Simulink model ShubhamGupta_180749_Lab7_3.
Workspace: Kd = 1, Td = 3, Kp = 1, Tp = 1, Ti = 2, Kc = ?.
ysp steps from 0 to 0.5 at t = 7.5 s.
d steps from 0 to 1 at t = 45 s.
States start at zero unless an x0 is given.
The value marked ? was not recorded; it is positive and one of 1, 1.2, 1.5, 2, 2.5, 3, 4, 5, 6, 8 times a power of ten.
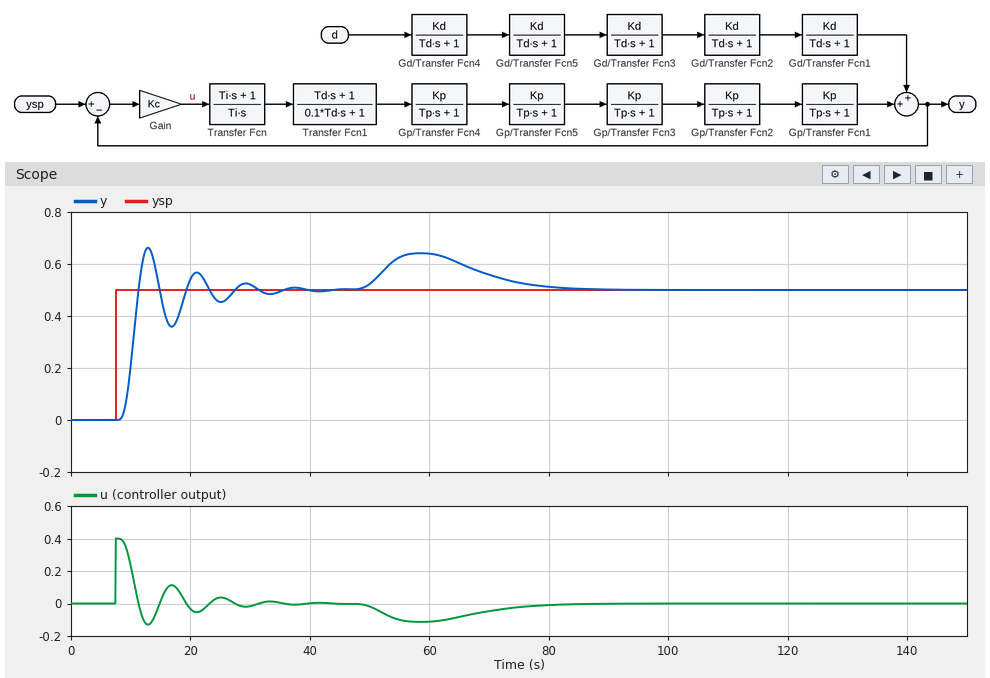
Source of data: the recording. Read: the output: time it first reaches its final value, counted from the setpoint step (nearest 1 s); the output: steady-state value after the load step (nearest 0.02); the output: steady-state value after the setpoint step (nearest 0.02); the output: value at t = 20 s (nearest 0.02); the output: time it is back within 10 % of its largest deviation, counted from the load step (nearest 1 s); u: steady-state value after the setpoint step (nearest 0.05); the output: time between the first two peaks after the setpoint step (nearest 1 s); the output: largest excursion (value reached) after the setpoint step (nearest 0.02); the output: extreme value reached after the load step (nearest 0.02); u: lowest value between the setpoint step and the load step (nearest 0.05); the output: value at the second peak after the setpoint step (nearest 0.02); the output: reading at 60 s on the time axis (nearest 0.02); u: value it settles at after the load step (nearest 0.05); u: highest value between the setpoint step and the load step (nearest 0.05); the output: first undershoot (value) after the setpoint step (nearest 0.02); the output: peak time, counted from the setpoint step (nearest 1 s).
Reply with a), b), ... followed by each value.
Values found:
a) 4 s
b) 0.50
c) 0.50
d) 0.54
e) 34 s
f) 0.00
g) 8 s
h) 0.66
i) 0.64
j) -0.15
k) 0.56
l) 0.64
m) 0.00
n) 0.40
o) 0.36
p) 5 s
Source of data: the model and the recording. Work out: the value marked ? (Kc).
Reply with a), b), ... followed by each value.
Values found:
a) 0.8
